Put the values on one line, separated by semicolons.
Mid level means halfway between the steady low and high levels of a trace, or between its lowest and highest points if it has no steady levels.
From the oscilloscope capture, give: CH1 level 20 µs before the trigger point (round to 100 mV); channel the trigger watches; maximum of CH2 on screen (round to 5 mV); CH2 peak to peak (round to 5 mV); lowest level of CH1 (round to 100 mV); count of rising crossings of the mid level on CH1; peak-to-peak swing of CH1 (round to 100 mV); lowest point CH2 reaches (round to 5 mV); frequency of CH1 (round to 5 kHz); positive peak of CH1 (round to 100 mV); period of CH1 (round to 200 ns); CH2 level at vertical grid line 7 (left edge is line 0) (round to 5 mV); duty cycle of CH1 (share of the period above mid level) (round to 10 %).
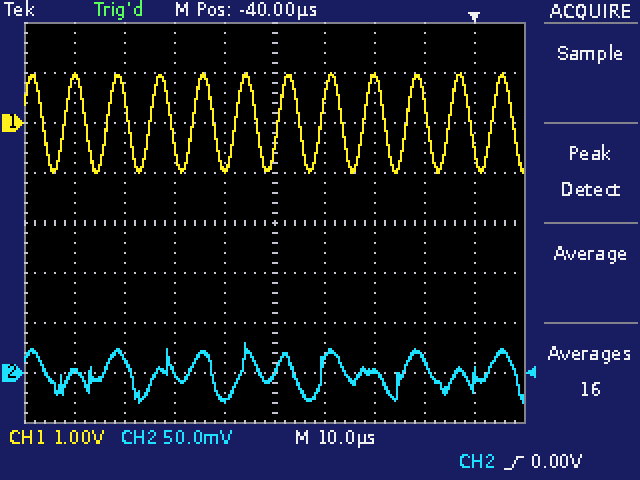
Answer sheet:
900 mV; CH2; 30 mV; 60 mV; -1.0 V; 11; 2.0 V; -30 mV; 115 kHz; 1.0 V; 8.6 µs; 0 mV; 50 %
